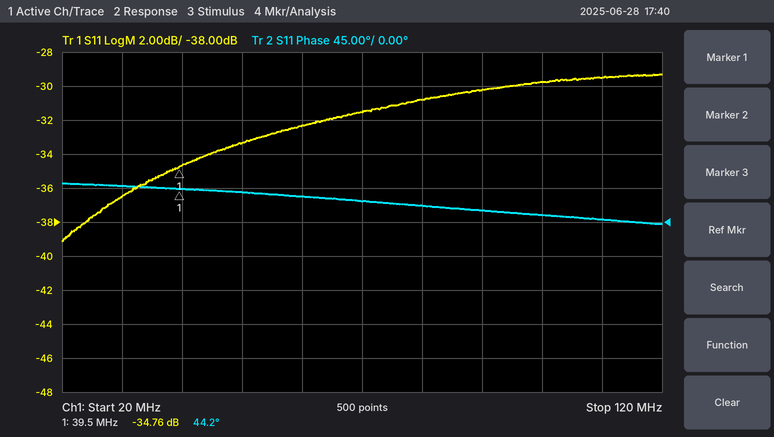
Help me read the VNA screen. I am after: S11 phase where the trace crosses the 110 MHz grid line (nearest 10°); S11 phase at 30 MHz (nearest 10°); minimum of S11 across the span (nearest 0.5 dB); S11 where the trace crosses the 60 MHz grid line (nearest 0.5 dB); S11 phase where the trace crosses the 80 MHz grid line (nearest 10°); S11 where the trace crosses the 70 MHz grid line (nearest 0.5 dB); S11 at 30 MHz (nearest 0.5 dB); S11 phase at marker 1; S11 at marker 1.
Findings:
0°
50°
-39.0 dB
-32.5 dB
20°
-31.5 dB
-36.5 dB
44.2°
-34.76 dB
